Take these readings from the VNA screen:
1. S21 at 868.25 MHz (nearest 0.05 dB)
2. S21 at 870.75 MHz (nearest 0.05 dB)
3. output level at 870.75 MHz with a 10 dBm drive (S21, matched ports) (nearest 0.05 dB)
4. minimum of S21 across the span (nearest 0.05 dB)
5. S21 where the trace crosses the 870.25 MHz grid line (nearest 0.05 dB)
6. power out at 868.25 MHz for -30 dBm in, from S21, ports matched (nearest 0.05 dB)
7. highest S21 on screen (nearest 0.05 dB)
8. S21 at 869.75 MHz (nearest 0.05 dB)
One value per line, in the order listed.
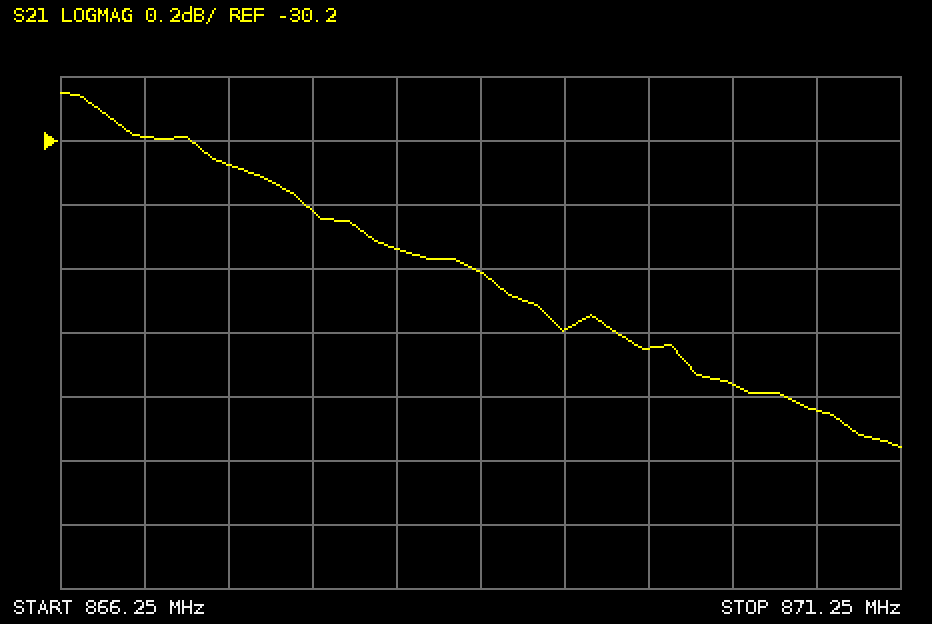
-30.55 dB
-31.05 dB
-21.05 dBm
-31.15 dB
-30.95 dB
-60.55 dBm
-30.05 dB
-30.85 dB
